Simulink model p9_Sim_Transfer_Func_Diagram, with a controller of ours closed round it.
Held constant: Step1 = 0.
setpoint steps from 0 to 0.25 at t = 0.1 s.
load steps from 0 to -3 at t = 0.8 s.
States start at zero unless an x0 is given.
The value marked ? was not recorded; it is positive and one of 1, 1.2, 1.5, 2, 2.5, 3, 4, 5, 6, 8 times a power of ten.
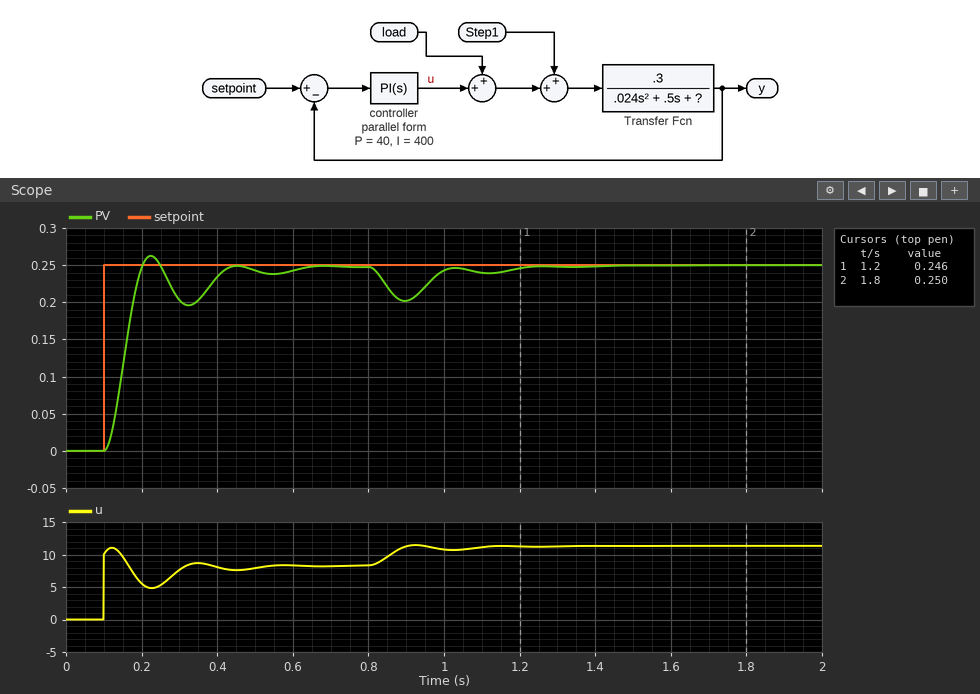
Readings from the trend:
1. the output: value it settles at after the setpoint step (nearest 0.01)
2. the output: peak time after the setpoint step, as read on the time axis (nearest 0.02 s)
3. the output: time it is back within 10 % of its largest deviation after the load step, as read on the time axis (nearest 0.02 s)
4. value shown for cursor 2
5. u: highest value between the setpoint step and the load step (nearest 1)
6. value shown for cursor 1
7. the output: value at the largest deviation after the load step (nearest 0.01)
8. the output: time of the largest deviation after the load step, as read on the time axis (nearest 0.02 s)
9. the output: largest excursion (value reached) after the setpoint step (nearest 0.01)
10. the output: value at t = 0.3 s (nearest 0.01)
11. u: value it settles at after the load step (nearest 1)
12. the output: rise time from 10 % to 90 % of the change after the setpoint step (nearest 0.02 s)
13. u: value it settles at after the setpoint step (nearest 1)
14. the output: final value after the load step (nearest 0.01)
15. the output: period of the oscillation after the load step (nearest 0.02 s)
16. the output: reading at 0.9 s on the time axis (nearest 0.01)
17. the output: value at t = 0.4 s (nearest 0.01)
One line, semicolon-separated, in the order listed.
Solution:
0.25; 0.22 s; 1.20 s; 0.250; 11; 0.246; 0.20; 0.90 s; 0.26; 0.20; 11; 0.06 s; 8; 0.25; 0.22 s; 0.20; 0.23
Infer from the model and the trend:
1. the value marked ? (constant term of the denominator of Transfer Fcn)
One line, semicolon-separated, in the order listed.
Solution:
10
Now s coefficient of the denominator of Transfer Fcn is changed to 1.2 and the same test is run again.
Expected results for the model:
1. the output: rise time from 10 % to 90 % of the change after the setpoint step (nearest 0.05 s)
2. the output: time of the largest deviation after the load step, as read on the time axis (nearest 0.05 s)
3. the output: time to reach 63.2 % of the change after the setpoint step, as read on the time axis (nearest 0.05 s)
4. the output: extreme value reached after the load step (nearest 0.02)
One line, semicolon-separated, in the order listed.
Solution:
0.15 s; 0.90 s; 0.20 s; 0.22
